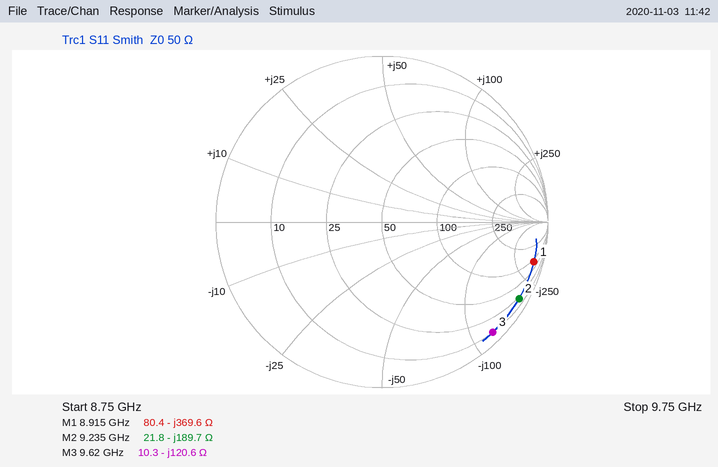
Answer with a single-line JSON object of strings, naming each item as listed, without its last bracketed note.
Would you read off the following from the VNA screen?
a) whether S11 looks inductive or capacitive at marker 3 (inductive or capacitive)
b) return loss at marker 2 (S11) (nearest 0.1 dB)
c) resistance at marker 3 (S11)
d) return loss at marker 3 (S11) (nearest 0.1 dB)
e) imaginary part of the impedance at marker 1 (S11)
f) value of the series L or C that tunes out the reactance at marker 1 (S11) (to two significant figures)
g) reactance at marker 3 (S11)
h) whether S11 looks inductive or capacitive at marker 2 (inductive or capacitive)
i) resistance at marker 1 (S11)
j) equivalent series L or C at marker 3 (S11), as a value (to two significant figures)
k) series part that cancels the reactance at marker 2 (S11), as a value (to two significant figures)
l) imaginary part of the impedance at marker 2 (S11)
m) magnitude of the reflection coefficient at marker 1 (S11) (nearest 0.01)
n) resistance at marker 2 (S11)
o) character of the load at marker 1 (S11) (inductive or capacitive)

{"whether S11 looks inductive or capacitive at marker 3": "capacitive", "return loss at marker 2 (S11)": "0.5 dB", "resistance at marker 3": "10.3 Ω", "return loss at marker 3 (S11)": "0.5 dB", "imaginary part of the impedance at marker 1": "-369.6 Ω", "value of the series L or C that tunes out the reactance at marker 1 (S11)": "6.6 nH", "reactance at marker 3": "-120.6 Ω", "whether S11 looks inductive or capacitive at marker 2": "capacitive", "resistance at marker 1": "80.4 Ω", "equivalent series L or C at marker 3 (S11), as a value": "140 fF", "series part that cancels the reactance at marker 2 (S11), as a value": "3.3 nH", "imaginary part of the impedance at marker 2": "-189.7 Ω", "magnitude of the reflection coefficient at marker 1 (S11)": "0.95", "resistance at marker 2": "21.8 Ω", "character of the load at marker 1 (S11)": "capacitive"}
